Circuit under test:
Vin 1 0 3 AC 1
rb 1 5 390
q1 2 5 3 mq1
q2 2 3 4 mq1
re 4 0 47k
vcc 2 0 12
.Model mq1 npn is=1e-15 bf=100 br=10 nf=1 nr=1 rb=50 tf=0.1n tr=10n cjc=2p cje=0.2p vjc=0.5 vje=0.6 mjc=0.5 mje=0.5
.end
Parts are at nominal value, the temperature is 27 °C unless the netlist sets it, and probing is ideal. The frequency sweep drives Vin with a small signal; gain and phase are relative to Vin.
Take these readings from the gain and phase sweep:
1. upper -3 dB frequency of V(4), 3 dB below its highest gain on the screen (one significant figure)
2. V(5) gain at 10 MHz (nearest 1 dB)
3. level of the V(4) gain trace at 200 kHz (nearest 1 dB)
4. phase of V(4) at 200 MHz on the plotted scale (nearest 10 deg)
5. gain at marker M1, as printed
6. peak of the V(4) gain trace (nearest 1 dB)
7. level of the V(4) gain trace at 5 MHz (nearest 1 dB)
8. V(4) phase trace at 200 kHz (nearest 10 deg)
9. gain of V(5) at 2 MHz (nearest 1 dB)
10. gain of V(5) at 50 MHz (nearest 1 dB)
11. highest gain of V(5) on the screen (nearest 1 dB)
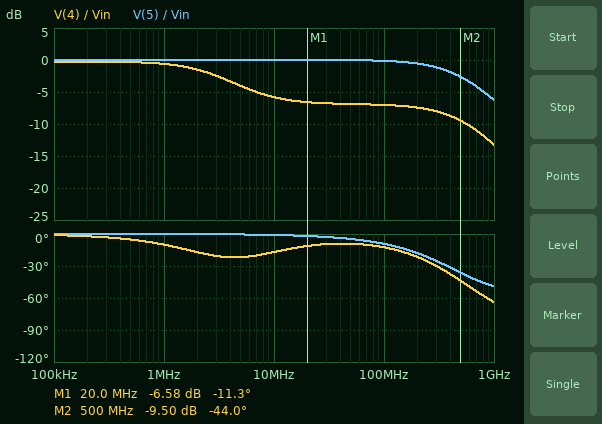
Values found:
4 MHz
0 dB
0 dB
-20 deg
-6.58 dB
0 dB
-4 dB
0 deg
0 dB
0 dB
0 dB
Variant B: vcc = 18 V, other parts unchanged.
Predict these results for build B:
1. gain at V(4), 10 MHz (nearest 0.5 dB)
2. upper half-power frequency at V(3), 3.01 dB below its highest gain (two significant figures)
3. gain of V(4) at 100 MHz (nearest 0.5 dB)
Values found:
-5.0 dB
4.9 MHz
-6.0 dB
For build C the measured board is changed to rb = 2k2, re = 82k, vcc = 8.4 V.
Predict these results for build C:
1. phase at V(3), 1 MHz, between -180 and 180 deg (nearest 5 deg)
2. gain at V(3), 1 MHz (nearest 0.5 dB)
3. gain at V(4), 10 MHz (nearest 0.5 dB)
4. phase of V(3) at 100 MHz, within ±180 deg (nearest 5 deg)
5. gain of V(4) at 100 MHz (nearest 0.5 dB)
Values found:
-20 deg
-1.5 dB
-7.5 dB
-50 deg
-11.5 dB
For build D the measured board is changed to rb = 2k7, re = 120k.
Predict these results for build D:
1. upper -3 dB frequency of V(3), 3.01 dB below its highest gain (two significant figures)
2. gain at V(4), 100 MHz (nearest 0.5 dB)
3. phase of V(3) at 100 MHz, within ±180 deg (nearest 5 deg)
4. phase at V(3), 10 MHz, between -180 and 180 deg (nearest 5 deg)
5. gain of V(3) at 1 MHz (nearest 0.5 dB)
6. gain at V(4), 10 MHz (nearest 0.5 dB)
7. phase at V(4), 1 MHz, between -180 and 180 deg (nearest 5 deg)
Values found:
1.6 MHz
-10.5 dB
-50 deg
-15 deg
-2.0 dB
-7.0 dB
-20 deg
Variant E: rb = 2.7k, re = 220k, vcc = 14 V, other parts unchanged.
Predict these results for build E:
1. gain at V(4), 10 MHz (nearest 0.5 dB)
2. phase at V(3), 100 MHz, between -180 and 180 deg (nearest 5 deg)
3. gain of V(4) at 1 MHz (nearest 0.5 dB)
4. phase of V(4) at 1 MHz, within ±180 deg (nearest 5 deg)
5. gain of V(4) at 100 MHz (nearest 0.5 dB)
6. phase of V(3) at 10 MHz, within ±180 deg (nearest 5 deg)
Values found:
-6.5 dB
-45 deg
-3.5 dB
-20 deg
-10.0 dB
-10 deg
